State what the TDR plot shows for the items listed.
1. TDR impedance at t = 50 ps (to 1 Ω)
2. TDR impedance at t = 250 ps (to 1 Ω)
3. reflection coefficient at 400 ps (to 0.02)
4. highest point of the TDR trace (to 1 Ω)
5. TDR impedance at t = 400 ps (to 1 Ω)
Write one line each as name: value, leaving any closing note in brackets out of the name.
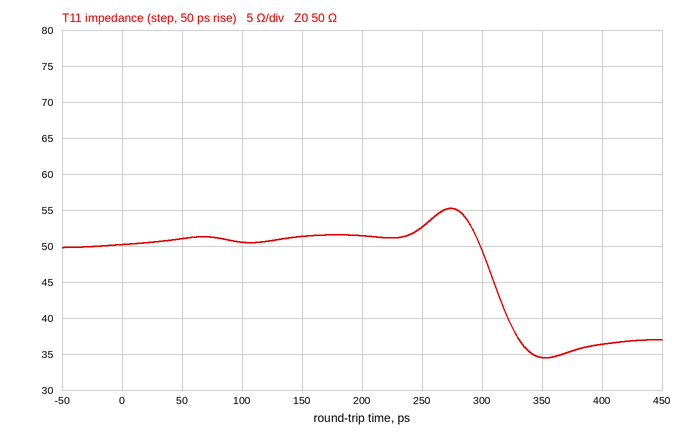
TDR impedance at t = 50 ps: 51 Ω
TDR impedance at t = 250 ps: 53 Ω
reflection coefficient at 400 ps: -0.16
highest point of the TDR trace: 55 Ω
TDR impedance at t = 400 ps: 36 Ω
